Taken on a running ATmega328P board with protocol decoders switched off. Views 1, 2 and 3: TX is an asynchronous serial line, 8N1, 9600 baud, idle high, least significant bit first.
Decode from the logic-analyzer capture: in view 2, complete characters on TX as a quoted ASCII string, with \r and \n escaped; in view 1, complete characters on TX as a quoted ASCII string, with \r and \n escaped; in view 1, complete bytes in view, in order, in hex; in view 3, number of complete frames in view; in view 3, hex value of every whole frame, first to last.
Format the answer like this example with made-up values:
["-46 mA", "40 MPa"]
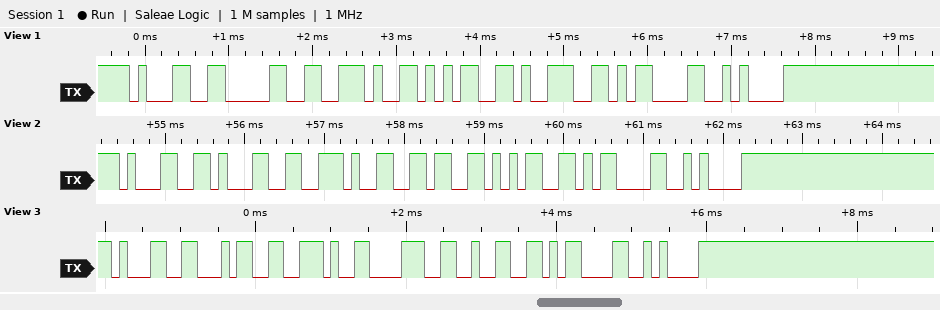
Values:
["\"11.65\\r\\n\"", "\"10.59\\r\\n\"", "0x31 0x30 0x2E 0x35 0x39 0x0D 0x0A", "7", "31 34 2E 38 32 0D 0A"]
